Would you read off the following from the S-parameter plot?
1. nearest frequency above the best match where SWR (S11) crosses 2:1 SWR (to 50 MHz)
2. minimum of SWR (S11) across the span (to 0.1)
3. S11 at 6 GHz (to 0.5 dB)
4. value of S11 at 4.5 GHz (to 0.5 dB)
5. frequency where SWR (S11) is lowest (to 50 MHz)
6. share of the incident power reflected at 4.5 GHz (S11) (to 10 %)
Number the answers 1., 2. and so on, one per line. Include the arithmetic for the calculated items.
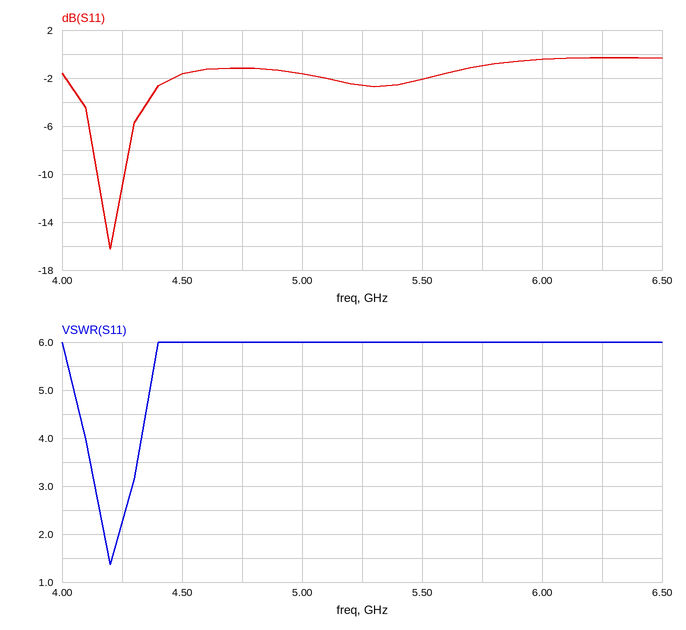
1. 4.25 GHz
2. 1.4
3. -0.5 dB
4. -1.5 dB
5. 4.20 GHz
6. 10^(-1.5/10) ≈ 70.8 %, so 70 % to the nearest 10 %
